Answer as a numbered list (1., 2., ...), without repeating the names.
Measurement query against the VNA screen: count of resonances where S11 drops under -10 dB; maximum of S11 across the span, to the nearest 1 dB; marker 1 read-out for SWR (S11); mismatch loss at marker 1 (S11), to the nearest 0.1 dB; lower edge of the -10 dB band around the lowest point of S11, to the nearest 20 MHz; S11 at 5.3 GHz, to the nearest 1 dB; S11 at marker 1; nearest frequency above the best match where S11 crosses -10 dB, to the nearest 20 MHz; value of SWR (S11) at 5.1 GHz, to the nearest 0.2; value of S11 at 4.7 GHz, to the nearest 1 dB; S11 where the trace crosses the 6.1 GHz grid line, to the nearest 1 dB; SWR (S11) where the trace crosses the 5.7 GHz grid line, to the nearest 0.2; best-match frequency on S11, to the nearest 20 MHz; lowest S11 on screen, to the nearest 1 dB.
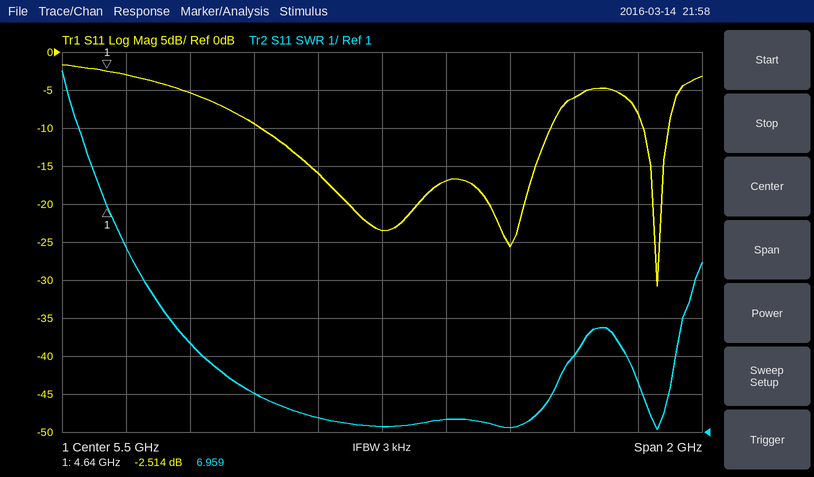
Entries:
1. 3
2. -2 dB
3. 6.959
4. 3.6 dB
5. 6.32 GHz
6. -16 dB
7. -2.514 dB
8. 6.40 GHz
9. 2.0
10. -3 dB
11. -6 dB
12. 1.4
13. 6.36 GHz
14. -31 dB
